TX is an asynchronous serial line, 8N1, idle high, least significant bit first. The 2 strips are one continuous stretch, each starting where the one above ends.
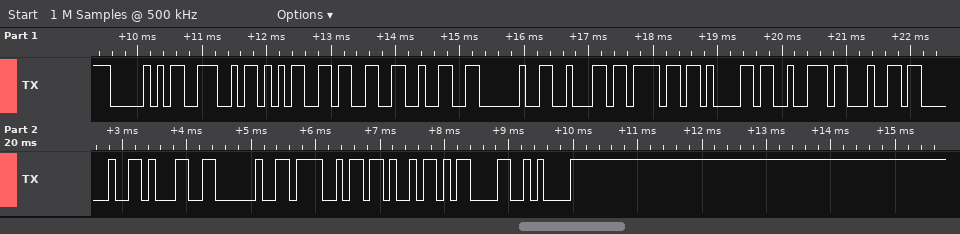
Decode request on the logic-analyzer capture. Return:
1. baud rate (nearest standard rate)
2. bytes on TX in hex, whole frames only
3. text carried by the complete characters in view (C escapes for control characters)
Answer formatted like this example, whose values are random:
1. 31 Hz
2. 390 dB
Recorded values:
1. 9600 baud
2. 50 4E 35 33 32 20 62 6F 61 72 64 20 31 20 4F 4B 0D 0A
3. "PN532 board 1 OK\r\n"
